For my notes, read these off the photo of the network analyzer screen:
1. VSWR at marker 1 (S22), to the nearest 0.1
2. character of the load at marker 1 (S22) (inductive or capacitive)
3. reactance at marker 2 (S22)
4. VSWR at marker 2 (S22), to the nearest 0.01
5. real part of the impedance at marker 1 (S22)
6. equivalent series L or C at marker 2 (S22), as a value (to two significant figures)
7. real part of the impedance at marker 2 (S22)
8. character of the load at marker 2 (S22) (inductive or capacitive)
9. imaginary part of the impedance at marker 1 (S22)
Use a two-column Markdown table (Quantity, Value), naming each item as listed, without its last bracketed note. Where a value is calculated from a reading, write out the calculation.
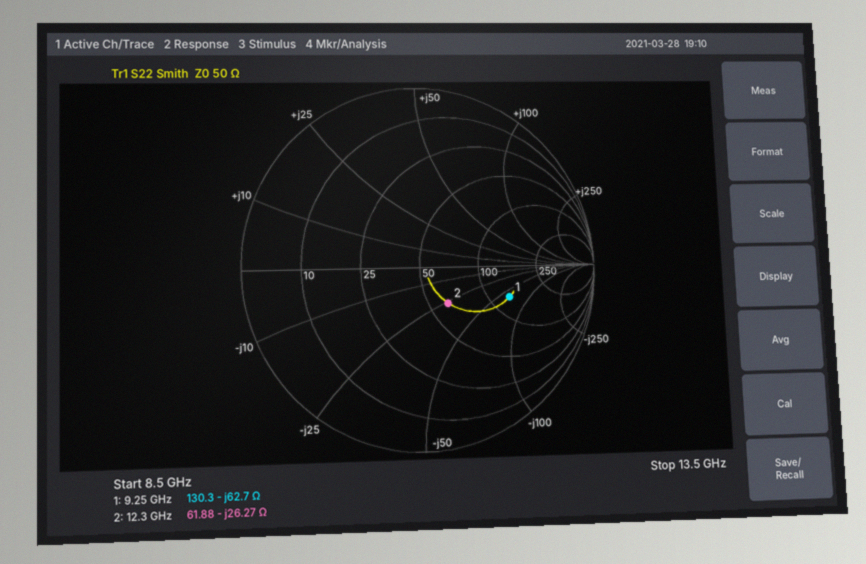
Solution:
| Quantity | Value |
|---|---|
| VSWR at marker 1 (S22), to the nearest 0.1 | 3.3 |
| character of the load at marker 1 (S22) | capacitive |
| reactance at marker 2 | -26.27 Ω |
| VSWR at marker 2 (S22), to the nearest 0.01 | 1.67 |
| real part of the impedance at marker 1 | 130.3 Ω |
| equivalent series L or C at marker 2 (S22), as a value | C = 1/(2π × 12.3 GHz × 26.27 Ω) ≈ 493 fF, so 490 fF to two significant figures |
| real part of the impedance at marker 2 | 61.88 Ω |
| character of the load at marker 2 (S22) | capacitive |
| imaginary part of the impedance at marker 1 | -62.7 Ω |
